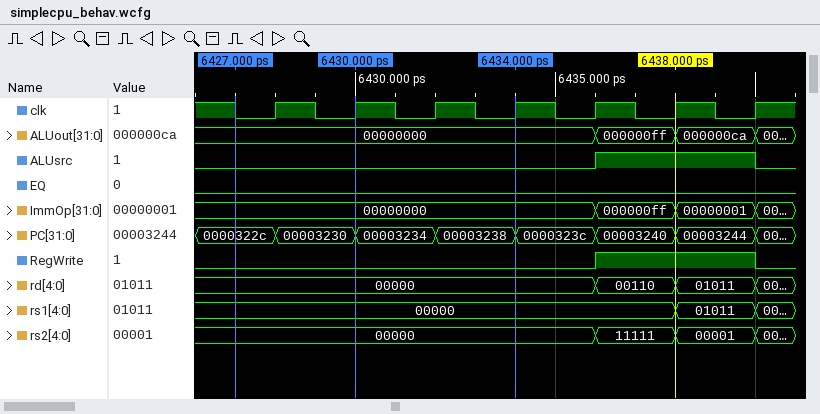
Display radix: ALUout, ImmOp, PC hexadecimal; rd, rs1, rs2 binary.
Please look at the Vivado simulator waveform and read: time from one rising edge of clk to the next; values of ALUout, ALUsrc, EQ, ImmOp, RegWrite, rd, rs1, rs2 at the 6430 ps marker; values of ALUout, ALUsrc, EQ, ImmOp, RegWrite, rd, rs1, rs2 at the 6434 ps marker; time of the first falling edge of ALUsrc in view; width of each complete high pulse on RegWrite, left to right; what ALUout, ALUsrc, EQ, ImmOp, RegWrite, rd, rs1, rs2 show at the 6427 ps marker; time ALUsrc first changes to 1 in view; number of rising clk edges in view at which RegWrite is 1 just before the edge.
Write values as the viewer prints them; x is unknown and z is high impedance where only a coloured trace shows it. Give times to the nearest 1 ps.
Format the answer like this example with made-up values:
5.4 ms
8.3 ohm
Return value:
2 ps
ALUout=00000000, ALUsrc=0, EQ=0, ImmOp=00000000, RegWrite=0, rd=00000, rs1=00000, rs2=00000
ALUout=00000000, ALUsrc=0, EQ=0, ImmOp=00000000, RegWrite=0, rd=00000, rs1=00000, rs2=00000
6440 ps
4 ps
ALUout=00000000, ALUsrc=0, EQ=0, ImmOp=00000000, RegWrite=0, rd=00000, rs1=00000, rs2=00000
6436 ps
2
